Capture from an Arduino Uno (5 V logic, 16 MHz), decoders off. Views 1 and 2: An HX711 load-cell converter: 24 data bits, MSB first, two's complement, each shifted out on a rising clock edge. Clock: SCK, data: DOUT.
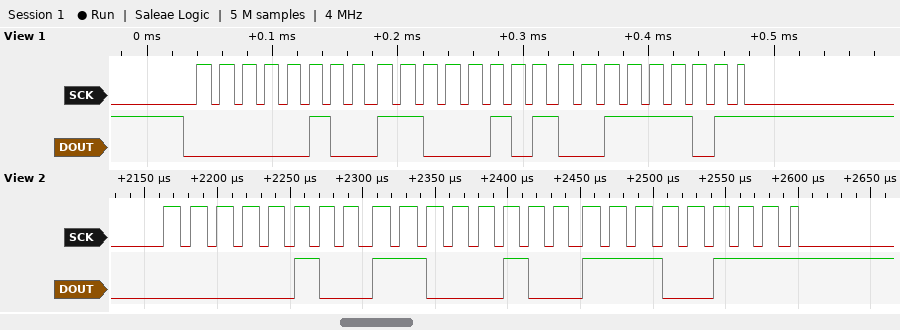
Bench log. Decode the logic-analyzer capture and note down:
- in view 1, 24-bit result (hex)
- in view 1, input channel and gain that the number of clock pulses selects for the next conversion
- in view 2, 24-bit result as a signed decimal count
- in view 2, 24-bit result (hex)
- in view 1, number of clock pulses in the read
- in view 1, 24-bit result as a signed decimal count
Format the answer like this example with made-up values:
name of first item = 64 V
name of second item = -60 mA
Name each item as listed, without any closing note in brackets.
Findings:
in view 1, 24-bit result = 0x04C53D
in view 1, input channel and gain that the number of clock pulses selects for the next conversion = channel A, gain 128
in view 2, 24-bit result as a signed decimal count = 312551
in view 2, 24-bit result = 0x04C4E7
in view 1, number of clock pulses in the read = 25
in view 1, 24-bit result as a signed decimal count = 312637
